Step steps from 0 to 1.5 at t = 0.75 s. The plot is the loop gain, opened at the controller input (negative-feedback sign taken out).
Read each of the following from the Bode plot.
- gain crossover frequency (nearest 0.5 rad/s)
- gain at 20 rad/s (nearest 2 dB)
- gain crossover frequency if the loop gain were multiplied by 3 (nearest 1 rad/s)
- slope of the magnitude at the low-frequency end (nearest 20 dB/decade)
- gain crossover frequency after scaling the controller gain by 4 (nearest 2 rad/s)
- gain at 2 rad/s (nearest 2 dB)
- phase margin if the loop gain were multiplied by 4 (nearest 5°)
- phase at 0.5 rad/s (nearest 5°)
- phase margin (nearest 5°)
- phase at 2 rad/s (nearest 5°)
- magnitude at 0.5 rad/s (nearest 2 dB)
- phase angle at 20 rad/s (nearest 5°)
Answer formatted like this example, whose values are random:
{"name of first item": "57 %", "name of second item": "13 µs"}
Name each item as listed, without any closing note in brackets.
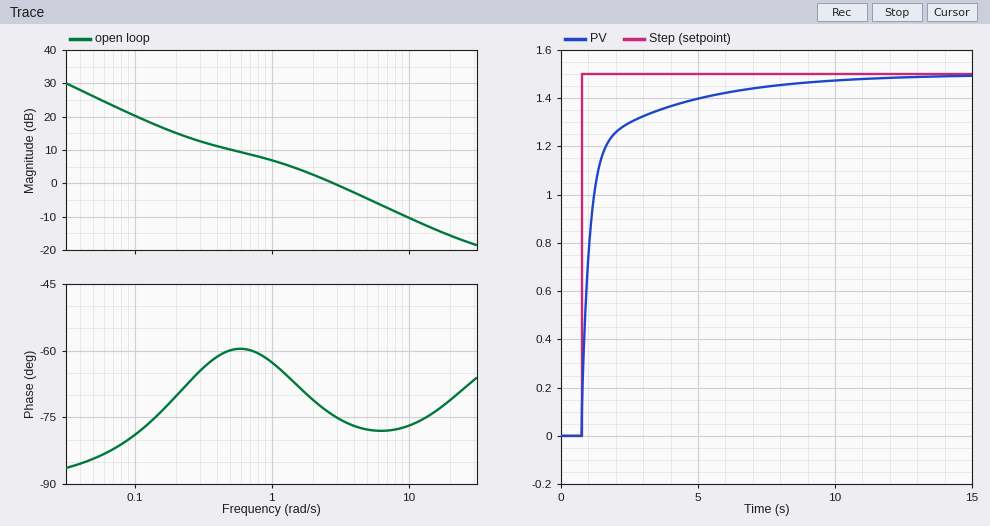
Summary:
{"gain crossover frequency": "3.0 rad/s", "gain at 20 rad/s": "-16 dB", "gain crossover frequency if the loop gain were multiplied by 3": "9 rad/s", "slope of the magnitude at the low-frequency end": "-20 dB/decade", "gain crossover frequency after scaling the controller gain by 4": "12 rad/s", "gain at 2 rad/s": "2 dB", "phase margin if the loop gain were multiplied by 4": "105°", "phase at 0.5 rad/s": "-60°", "phase margin": "105°", "phase at 2 rad/s": "-70°", "magnitude at 0.5 rad/s": "10 dB", "phase angle at 20 rad/s": "-70°"}
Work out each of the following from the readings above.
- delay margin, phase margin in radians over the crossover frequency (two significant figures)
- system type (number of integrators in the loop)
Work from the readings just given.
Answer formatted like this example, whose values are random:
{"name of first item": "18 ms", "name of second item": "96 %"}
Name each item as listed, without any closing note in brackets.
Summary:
{"delay margin, phase margin in radians over the crossover frequency": "0.61 s", "system type": "1"}
